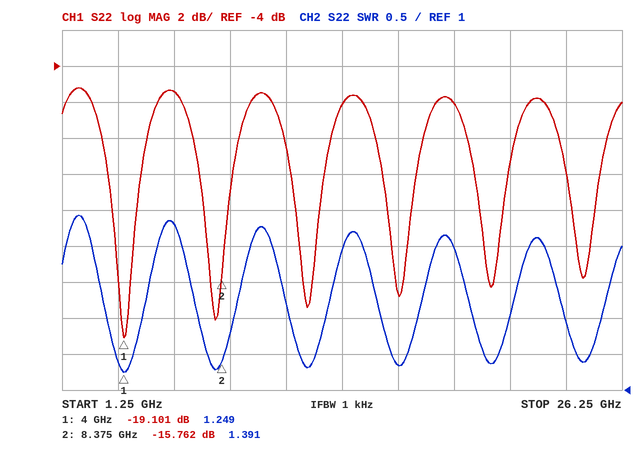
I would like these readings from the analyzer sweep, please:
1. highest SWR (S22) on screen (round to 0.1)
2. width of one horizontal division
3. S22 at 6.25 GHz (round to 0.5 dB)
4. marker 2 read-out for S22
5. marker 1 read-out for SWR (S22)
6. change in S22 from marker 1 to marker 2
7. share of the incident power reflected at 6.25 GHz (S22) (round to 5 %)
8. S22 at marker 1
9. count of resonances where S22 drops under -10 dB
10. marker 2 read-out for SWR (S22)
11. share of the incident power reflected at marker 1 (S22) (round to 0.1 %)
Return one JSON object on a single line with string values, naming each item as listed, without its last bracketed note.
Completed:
{"highest SWR (S22) on screen": "3.4", "width of one horizontal division": "2.5 GHz", "S22 at 6.25 GHz": "-5.5 dB", "marker 2 read-out for S22": "-15.762 dB", "marker 1 read-out for SWR": "1.249", "change in S22 from marker 1 to marker 2": "3.339 dB", "share of the incident power reflected at 6.25 GHz (S22)": "30 %", "S22 at marker 1": "-19.101 dB", "count of resonances where S22 drops under -10 dB": "6", "marker 2 read-out for SWR": "1.391", "share of the incident power reflected at marker 1 (S22)": "1.2 %"}
